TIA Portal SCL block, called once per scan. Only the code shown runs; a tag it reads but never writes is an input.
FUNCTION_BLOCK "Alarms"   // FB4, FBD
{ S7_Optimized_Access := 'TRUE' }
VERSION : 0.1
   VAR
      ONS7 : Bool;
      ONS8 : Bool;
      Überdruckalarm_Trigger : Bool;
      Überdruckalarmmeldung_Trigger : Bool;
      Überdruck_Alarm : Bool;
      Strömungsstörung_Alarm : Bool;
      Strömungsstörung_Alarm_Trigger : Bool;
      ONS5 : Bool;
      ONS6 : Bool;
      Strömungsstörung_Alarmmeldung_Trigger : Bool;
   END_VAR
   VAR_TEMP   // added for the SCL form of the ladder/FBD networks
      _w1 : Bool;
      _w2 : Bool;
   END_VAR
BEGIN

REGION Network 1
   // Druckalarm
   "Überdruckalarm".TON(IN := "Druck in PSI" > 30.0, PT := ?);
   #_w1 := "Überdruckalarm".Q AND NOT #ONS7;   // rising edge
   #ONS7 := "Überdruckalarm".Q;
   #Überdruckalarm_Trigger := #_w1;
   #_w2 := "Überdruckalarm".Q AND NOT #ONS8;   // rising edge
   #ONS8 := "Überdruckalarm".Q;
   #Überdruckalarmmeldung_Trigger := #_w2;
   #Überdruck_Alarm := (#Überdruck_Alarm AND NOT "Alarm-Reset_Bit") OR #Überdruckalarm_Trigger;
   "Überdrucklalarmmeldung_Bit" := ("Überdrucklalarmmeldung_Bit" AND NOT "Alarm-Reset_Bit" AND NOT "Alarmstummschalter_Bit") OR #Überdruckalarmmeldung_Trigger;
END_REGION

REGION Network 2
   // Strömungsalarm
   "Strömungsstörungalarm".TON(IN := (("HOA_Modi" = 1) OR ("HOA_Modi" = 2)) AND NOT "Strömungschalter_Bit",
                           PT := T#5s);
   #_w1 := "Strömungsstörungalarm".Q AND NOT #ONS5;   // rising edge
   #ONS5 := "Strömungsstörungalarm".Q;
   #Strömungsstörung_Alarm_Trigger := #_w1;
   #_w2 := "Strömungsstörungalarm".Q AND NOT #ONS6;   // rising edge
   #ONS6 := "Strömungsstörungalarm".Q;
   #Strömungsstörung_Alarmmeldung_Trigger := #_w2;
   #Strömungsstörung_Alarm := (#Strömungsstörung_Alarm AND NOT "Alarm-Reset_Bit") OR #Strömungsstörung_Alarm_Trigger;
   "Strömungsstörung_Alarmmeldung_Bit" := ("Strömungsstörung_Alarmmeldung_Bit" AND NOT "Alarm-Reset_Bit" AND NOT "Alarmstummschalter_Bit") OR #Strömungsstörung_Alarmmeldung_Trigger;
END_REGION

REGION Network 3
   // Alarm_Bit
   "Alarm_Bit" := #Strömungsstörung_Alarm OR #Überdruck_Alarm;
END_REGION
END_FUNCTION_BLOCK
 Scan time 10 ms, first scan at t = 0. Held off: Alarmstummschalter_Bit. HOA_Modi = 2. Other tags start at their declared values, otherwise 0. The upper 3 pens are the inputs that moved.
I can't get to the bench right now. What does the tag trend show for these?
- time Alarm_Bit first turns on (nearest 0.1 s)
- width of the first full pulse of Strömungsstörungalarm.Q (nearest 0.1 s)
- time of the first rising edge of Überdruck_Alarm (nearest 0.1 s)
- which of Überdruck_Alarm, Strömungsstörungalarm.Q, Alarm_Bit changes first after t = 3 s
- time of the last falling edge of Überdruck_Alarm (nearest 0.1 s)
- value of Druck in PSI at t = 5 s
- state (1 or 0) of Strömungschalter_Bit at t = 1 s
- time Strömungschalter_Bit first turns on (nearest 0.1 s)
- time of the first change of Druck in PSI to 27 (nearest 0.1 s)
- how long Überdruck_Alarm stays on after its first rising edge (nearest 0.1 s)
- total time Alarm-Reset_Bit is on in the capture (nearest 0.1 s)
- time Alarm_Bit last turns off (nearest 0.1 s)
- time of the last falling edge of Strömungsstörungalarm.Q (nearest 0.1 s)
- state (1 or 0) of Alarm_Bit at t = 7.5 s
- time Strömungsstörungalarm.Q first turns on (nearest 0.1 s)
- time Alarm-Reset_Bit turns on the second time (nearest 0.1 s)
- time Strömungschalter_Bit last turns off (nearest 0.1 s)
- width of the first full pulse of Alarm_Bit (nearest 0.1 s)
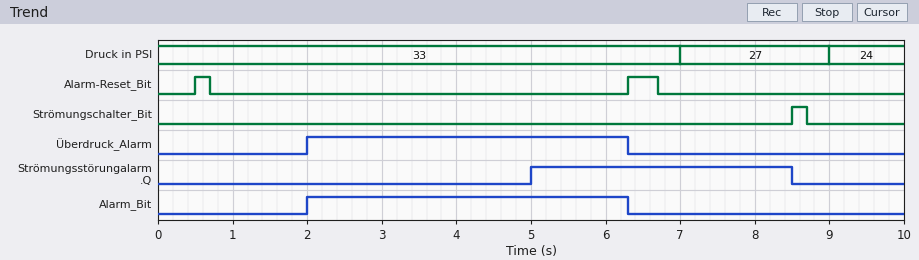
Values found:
2.0 s
3.5 s
2.0 s
Strömungsstörungalarm.Q
6.3 s
33
0
8.5 s
7.0 s
4.3 s
0.6 s
6.3 s
8.5 s
0
5.0 s
6.3 s
8.7 s
4.3 s
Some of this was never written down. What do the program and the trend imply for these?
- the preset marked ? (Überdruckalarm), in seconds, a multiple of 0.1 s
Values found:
2.0 s
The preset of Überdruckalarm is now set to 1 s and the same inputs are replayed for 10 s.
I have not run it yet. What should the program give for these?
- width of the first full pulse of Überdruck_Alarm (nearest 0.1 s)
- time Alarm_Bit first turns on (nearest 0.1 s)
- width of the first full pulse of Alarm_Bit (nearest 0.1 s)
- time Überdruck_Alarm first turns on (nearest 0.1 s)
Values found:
5.3 s
1.0 s
5.3 s
1.0 s
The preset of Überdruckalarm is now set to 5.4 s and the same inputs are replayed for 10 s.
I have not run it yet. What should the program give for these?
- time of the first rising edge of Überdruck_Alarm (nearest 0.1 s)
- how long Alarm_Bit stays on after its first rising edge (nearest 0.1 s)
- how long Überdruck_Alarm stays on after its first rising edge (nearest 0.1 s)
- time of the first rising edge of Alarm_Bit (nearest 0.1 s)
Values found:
5.4 s
1.3 s
0.9 s
5.0 s
